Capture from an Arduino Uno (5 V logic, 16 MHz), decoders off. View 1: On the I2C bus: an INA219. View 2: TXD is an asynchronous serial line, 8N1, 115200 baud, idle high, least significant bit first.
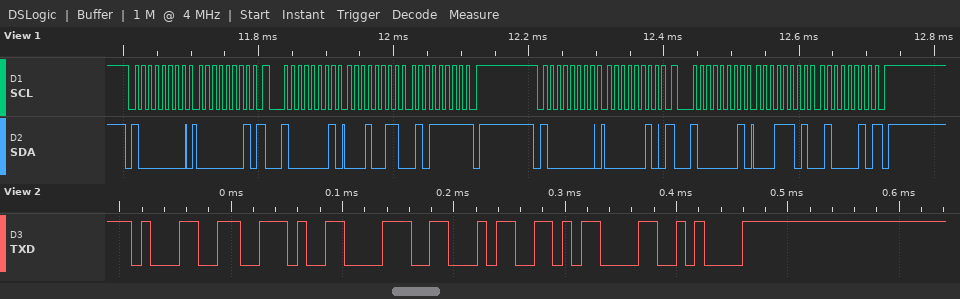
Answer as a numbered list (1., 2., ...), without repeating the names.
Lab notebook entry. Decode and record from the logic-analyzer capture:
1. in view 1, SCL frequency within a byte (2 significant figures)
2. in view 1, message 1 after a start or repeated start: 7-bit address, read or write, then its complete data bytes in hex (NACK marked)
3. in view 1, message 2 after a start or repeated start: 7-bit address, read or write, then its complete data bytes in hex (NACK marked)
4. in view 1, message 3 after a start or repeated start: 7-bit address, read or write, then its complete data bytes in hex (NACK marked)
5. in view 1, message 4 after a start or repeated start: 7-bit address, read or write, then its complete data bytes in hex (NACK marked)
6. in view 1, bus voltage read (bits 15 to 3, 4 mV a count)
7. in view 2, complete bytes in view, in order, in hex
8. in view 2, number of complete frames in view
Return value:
1. 100 kHz
2. 0x40 write: 01
3. 0x40 read: 13 5F NACK
4. 0x40 write: 02
5. 0x40 read: 1D 42 NACK
6. 3.744 V
7. 31 2E 38 34 0D 0A
8. 6
